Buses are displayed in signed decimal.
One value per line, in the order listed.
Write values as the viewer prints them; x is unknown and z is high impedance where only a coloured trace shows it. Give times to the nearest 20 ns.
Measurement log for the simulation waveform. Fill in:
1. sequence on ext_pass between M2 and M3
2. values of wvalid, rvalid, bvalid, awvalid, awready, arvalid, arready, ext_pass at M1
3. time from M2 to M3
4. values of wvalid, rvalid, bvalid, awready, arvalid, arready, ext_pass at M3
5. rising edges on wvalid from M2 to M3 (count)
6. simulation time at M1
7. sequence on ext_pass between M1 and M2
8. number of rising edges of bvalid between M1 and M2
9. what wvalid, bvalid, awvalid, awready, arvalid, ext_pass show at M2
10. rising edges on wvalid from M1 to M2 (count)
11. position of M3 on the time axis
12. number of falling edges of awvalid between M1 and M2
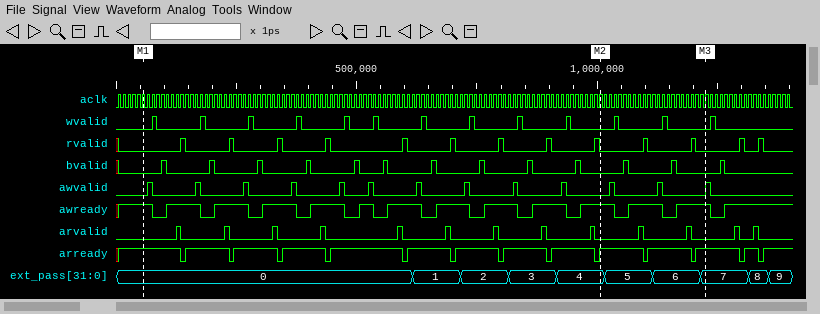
4, 5, 6, 7
wvalid=0, rvalid=0, bvalid=0, awvalid=0, awready=1, arvalid=0, arready=1, ext_pass=0
220 ns
wvalid=0, rvalid=0, bvalid=0, awready=1, arvalid=0, arready=1, ext_pass=7
2
60 ns
0, 1, 2, 3, 4
10
wvalid=0, bvalid=0, awvalid=0, awready=1, arvalid=0, ext_pass=4
10
1220 ns
10
